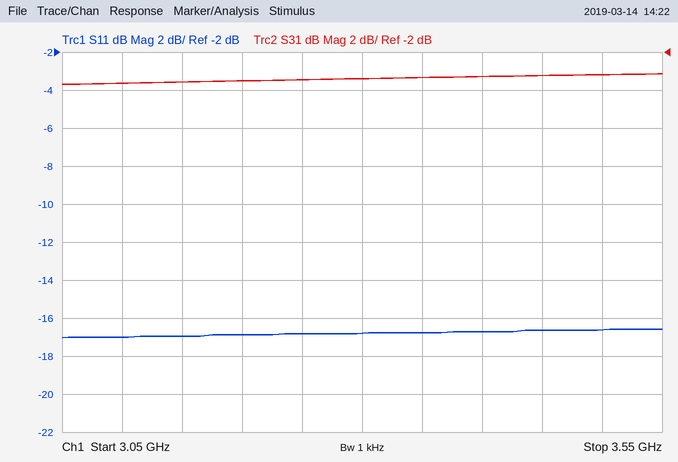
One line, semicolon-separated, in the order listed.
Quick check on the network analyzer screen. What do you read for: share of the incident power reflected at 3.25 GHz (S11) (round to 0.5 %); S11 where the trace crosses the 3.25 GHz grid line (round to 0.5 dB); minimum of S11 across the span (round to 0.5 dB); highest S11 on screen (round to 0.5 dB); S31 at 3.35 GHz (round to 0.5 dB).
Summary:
2.0 %; -17.0 dB; -17.0 dB; -16.5 dB; -3.5 dB
